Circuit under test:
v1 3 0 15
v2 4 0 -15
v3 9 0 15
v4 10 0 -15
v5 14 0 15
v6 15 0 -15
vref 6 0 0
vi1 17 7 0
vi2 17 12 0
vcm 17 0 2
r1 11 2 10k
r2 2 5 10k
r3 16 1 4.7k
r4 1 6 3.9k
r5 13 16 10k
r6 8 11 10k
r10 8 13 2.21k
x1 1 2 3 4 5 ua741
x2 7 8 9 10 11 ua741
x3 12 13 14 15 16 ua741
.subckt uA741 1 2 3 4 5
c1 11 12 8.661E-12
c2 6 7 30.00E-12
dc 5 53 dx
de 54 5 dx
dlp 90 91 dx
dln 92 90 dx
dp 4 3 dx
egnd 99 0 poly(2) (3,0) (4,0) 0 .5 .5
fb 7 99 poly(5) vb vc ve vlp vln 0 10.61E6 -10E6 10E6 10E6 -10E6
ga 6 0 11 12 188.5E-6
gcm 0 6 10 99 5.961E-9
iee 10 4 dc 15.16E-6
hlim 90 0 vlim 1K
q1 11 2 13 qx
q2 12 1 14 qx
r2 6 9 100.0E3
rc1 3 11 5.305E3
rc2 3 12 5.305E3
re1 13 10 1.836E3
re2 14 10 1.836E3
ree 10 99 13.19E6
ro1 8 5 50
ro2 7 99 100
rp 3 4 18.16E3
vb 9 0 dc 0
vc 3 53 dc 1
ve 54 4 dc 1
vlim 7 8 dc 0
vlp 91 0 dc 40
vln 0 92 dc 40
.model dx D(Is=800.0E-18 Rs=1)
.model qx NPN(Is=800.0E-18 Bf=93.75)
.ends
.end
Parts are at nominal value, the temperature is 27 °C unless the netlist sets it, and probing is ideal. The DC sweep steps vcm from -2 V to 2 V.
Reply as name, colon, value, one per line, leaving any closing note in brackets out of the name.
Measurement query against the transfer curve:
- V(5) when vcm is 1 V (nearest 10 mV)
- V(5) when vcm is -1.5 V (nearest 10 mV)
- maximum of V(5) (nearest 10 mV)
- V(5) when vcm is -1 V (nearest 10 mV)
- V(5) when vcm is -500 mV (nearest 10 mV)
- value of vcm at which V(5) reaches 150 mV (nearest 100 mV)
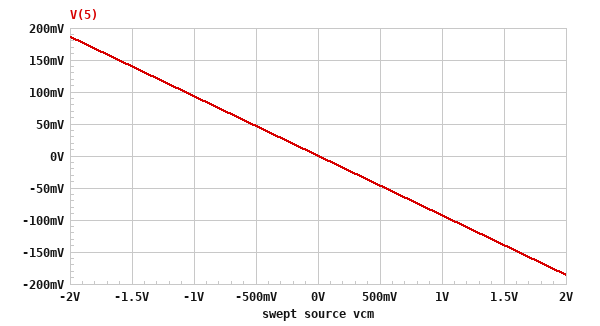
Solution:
V(5) when vcm is 1 V: -90 mV
V(5) when vcm is -1.5 V: 140 mV
maximum of V(5): 190 mV
V(5) when vcm is -1 V: 90 mV
V(5) when vcm is -500 mV: 50 mV
value of vcm at which V(5) reaches 150 mV: -1.6 V
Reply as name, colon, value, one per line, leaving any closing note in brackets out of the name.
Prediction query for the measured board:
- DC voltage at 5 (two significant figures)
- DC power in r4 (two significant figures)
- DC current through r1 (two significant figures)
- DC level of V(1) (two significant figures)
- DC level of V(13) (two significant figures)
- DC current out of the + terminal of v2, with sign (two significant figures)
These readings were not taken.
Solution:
DC voltage at 5: -190 mV
DC power in r4: 210 µW
DC current through r1: 110 µA
DC level of V(1): 910 mV
DC level of V(13): 2.0 V
DC current out of the + terminal of v2, with sign: -1.7 mA
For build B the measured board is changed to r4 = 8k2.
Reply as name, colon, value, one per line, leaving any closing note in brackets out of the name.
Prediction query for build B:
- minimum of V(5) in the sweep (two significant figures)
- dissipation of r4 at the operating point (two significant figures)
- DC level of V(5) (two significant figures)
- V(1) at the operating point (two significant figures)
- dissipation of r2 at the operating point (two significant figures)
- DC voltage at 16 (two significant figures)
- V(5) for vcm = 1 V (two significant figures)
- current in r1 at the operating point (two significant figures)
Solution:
minimum of V(5) in the sweep: -540 mV
dissipation of r4 at the operating point: 200 µW
DC level of V(5): 540 mV
V(1) at the operating point: 1.3 V
dissipation of r2 at the operating point: 53 µW
DC voltage at 16: 2.0 V
V(5) for vcm = 1 V: 270 mV
current in r1 at the operating point: 73 µA
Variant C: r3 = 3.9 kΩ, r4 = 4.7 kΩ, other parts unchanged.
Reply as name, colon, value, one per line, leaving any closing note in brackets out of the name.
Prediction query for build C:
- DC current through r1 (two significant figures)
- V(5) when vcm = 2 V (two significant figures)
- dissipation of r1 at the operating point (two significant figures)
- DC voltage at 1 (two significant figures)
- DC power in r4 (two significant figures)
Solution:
DC current through r1: 91 µA
V(5) when vcm = 2 V: 190 mV
dissipation of r1 at the operating point: 82 µW
DC voltage at 1: 1.1 V
DC power in r4: 250 µW
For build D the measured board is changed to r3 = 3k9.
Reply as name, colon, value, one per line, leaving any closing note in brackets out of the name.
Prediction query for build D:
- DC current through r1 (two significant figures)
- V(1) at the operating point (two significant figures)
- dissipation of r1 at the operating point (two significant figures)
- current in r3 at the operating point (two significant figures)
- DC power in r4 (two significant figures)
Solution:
DC current through r1: 100 µA
V(1) at the operating point: 1.0 V
dissipation of r1 at the operating point: 100 µW
current in r3 at the operating point: 260 µA
DC power in r4: 260 µW
